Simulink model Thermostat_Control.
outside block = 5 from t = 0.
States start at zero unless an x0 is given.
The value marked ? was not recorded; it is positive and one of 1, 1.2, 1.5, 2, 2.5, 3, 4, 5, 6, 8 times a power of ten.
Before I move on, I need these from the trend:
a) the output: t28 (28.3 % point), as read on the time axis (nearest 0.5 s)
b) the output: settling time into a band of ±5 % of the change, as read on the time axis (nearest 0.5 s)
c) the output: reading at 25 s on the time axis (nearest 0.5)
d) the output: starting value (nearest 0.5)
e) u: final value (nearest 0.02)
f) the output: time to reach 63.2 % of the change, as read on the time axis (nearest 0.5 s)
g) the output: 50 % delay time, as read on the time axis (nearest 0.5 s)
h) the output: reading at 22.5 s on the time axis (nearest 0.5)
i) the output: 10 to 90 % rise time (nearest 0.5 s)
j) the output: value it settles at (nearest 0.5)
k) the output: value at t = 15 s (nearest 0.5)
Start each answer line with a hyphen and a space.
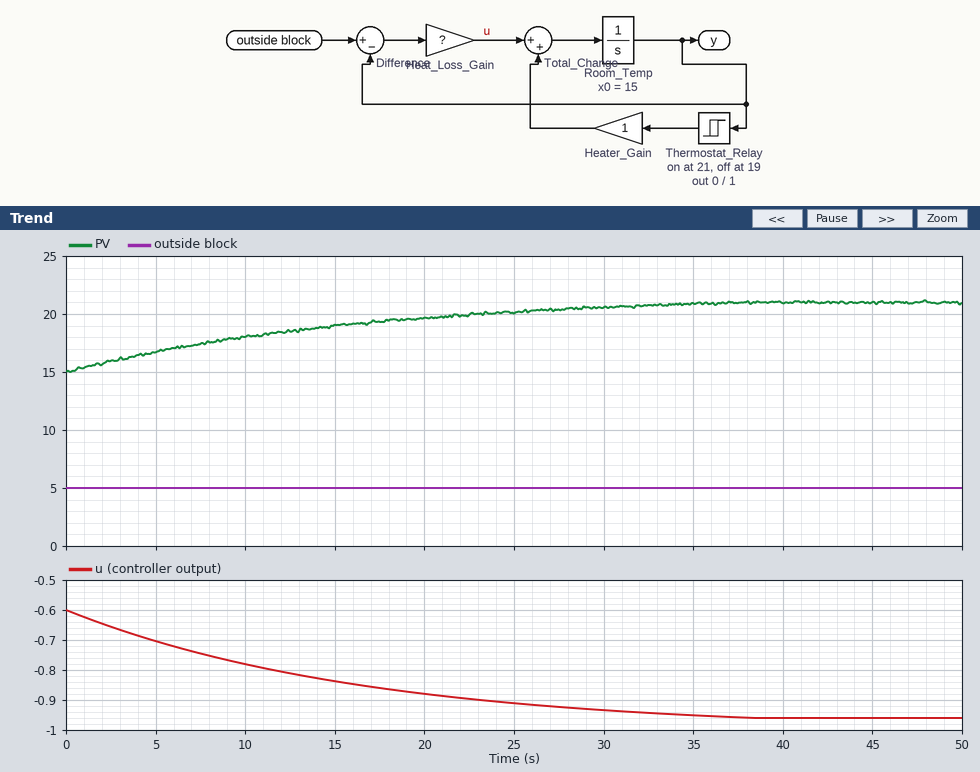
- 5.0 s
- 32.0 s
- 20.0
- 15.0
- -0.96
- 14.0 s
- 10.0 s
- 20.0
- 26.0 s
- 21.0
- 19.0
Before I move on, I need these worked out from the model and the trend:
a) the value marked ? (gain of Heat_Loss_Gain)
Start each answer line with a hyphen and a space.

- 0.06
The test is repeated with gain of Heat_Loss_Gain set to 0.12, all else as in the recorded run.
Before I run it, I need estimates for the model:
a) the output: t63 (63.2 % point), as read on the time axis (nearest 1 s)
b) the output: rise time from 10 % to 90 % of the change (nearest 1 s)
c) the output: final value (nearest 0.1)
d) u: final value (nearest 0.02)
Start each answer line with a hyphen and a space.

- 8 s
- 18 s
- 13.3
- -1.00
